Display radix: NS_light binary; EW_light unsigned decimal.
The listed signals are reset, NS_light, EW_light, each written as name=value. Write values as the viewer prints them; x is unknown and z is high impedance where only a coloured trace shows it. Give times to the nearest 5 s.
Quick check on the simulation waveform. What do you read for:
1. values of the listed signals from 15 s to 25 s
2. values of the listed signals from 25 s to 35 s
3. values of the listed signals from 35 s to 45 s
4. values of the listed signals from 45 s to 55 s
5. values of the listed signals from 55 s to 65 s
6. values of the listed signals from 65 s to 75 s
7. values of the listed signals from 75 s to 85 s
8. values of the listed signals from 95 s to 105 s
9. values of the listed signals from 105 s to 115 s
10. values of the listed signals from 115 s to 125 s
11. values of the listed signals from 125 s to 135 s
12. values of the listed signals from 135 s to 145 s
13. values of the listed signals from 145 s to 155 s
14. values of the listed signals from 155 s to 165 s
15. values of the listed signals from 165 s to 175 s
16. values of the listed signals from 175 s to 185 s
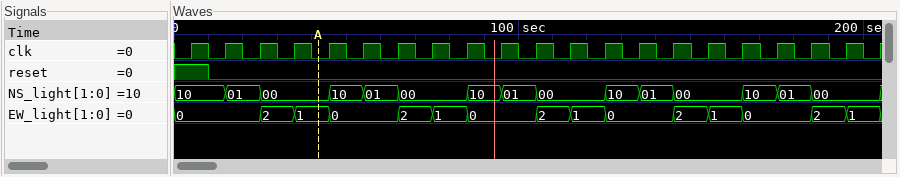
reset=0, NS_light=01, EW_light=0
reset=0, NS_light=00, EW_light=2
reset=0, NS_light=00, EW_light=1
reset=0, NS_light=10, EW_light=0
reset=0, NS_light=01, EW_light=0
reset=0, NS_light=00, EW_light=2
reset=0, NS_light=00, EW_light=1
reset=0, NS_light=01, EW_light=0
reset=0, NS_light=00, EW_light=2
reset=0, NS_light=00, EW_light=1
reset=0, NS_light=10, EW_light=0
reset=0, NS_light=01, EW_light=0
reset=0, NS_light=00, EW_light=2
reset=0, NS_light=00, EW_light=1
reset=0, NS_light=10, EW_light=0
reset=0, NS_light=01, EW_light=0
